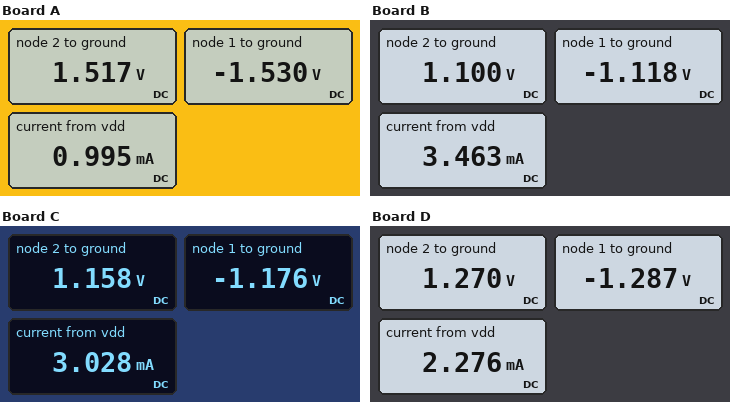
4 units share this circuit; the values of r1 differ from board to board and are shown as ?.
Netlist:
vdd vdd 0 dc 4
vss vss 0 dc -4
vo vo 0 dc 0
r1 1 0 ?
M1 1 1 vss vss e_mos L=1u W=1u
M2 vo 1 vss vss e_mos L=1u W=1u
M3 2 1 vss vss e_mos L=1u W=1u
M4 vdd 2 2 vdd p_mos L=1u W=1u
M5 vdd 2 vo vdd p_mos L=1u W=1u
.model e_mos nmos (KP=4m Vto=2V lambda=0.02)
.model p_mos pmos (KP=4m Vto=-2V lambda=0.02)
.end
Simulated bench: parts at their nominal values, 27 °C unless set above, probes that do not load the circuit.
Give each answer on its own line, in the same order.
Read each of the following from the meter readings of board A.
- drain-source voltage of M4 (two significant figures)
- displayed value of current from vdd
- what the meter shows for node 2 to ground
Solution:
2.5 V
0.995 mA
1.517 V
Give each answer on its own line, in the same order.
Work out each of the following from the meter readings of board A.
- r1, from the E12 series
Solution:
3.3 kΩ
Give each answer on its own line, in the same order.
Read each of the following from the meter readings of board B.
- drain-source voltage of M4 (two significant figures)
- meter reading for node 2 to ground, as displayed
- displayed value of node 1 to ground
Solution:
2.9 V
1.100 V
-1.118 V
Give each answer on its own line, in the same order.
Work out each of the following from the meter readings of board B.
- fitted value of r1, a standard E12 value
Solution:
680 Ω
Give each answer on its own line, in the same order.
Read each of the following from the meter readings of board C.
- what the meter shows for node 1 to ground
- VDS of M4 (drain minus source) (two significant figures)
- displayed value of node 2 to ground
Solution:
-1.176 V
2.8 V
1.158 V
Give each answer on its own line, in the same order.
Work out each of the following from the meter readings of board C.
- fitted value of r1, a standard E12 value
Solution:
820 Ω
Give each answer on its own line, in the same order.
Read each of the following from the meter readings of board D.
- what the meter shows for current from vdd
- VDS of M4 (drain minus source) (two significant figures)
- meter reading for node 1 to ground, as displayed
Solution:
2.276 mA
2.7 V
-1.287 V
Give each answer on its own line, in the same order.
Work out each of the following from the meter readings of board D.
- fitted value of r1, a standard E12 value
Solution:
1.2 kΩ
